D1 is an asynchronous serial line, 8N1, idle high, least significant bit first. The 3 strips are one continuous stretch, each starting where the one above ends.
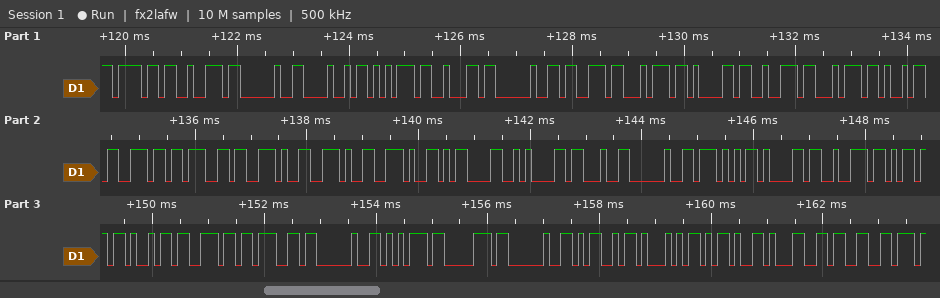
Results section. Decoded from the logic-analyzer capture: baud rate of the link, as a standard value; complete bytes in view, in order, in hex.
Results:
9600 baud
6F 72 20 48 75 62 20 73 74 61 72 74 69 6E 67 2E 2E 2E 0D 0A 23 20 57 61 72 6D 69 6E 67 20 75 70 20 4D 51 2D 31 33
